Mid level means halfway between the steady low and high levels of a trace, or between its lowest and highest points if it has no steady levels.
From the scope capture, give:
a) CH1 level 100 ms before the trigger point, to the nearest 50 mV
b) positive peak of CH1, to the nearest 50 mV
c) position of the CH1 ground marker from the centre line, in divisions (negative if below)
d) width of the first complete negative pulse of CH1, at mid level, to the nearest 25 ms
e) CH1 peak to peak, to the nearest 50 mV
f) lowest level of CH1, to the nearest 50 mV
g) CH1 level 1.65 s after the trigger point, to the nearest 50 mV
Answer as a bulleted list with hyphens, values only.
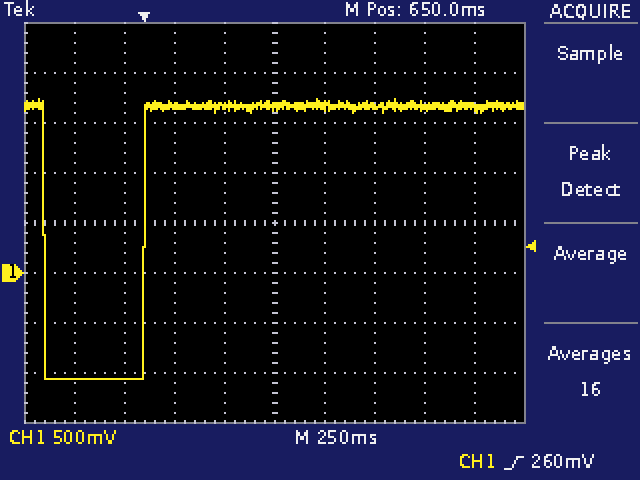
- -1.05 V
- 1.75 V
- -1.0 div
- 500 ms
- 2.80 V
- -1.05 V
- 1.65 V
